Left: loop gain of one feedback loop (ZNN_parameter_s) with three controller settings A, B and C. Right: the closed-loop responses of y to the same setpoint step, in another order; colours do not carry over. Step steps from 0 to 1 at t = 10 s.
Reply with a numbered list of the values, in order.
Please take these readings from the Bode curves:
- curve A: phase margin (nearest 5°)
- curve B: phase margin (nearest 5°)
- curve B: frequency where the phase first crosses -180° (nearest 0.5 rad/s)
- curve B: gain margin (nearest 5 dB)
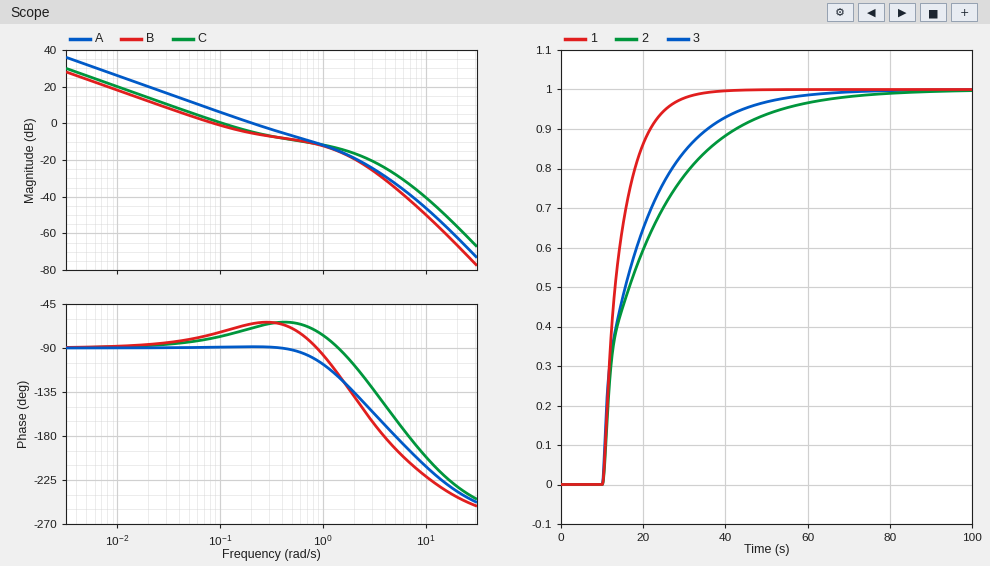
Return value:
1. 90°
2. 105°
3. 4.0 rad/s
4. 30 dB
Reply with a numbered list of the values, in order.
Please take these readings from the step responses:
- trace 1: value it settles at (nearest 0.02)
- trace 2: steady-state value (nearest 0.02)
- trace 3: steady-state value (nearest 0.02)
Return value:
1. 1.00
2. 1.00
3. 1.00
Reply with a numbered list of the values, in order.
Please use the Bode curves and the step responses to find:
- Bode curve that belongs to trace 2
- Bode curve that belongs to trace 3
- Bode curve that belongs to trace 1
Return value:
1. B
2. C
3. A
